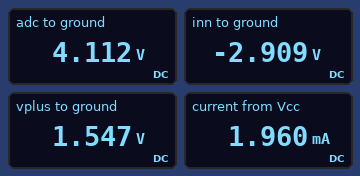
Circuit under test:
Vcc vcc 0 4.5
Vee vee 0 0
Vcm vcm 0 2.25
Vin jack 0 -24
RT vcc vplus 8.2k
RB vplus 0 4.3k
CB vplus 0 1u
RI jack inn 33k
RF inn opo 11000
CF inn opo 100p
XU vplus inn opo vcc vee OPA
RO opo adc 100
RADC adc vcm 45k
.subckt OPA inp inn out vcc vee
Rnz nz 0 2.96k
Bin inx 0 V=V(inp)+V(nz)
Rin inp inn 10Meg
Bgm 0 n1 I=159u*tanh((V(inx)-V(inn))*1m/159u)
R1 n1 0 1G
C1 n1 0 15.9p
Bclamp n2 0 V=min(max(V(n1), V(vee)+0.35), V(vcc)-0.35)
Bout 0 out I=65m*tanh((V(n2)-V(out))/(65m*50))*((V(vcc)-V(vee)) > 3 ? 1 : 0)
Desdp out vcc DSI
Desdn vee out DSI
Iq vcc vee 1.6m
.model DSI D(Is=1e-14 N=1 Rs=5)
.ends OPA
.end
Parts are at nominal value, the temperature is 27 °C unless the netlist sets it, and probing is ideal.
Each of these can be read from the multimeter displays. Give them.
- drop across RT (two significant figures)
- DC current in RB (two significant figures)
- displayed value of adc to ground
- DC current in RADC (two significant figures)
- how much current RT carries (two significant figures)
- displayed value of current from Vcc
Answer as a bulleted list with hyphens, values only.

- 3.0 V
- 360 µA
- 4.112 V
- 41 µA
- 360 µA
- 1.960 mA
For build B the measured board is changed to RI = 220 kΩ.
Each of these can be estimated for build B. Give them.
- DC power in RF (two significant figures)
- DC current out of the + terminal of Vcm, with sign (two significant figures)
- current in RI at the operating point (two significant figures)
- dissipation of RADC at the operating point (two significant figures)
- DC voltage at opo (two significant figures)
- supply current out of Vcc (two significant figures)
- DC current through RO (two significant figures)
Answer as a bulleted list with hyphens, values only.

- 150 µW
- -13 µA
- 120 µA
- 7.3 µW
- 2.8 V
- 2.0 mA
- 13 µA
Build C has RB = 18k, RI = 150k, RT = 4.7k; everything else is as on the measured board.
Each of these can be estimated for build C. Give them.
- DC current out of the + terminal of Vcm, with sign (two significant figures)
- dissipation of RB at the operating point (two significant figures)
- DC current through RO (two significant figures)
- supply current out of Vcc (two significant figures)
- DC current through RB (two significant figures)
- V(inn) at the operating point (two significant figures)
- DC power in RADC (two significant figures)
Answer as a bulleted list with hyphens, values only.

- -42 µA
- 710 µW
- 42 µA
- 1.8 mA
- 200 µA
- 2.2 V
- 79 µW
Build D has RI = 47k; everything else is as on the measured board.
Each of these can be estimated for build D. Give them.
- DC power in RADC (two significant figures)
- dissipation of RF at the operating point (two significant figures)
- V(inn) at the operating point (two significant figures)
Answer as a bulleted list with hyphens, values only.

- 78 µW
- 2.6 mW
- -1.2 V
